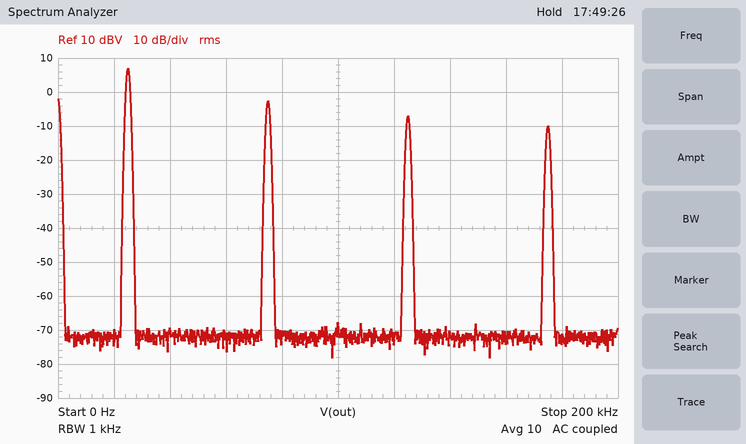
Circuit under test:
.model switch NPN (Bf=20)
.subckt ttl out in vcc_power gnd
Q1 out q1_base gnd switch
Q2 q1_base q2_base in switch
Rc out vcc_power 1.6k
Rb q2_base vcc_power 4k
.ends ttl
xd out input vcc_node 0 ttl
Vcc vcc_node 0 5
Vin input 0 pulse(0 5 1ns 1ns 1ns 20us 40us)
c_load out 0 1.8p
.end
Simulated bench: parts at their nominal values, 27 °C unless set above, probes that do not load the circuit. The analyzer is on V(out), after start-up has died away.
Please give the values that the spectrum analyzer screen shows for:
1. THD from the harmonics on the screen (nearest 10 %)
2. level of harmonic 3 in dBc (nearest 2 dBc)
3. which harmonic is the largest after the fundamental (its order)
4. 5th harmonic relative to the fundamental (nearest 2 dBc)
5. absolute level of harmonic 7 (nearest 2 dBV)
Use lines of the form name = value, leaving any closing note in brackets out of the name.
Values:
THD from the harmonics on the screen = 40 %
level of harmonic 3 in dBc = -10 dBc
which harmonic is the largest after the fundamental = 3
5th harmonic relative to the fundamental = -14 dBc
absolute level of harmonic 7 = -10 dBV
